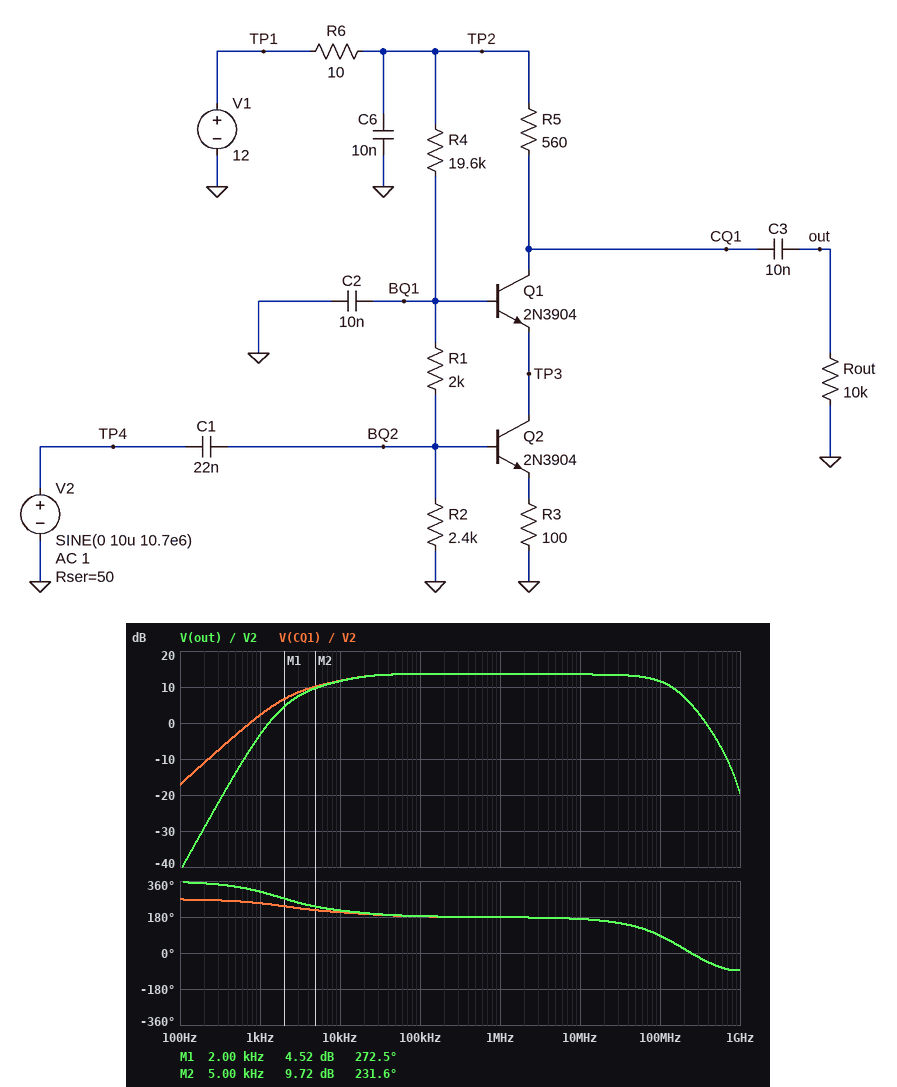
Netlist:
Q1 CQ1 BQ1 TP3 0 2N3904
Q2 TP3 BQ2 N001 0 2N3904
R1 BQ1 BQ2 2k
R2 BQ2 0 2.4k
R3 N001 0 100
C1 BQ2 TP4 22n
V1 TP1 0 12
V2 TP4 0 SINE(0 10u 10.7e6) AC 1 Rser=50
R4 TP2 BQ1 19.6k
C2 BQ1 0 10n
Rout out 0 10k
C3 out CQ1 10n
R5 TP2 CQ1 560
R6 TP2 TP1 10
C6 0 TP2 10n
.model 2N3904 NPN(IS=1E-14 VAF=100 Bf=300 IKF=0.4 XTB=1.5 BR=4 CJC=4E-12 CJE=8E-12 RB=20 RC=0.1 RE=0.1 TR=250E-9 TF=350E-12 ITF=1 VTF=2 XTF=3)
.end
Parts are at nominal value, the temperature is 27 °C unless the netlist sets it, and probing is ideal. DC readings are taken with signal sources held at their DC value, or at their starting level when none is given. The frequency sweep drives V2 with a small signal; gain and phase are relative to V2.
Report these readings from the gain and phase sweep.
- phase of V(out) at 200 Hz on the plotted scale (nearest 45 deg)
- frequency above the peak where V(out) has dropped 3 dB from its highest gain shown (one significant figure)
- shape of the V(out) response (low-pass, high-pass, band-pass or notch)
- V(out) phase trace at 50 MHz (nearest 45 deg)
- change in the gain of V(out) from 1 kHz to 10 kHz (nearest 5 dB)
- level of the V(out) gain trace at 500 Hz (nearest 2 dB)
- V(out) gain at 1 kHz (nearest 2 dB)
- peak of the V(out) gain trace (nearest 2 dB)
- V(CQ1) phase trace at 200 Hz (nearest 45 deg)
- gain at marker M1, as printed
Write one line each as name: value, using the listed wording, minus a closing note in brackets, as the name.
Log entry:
phase of V(out) at 200 Hz on the plotted scale: 360 deg
frequency above the peak where V(out) has dropped 3 dB from its highest gain shown: 100 MHz
shape of the V(out) response: band-pass
V(out) phase trace at 50 MHz: 135 deg
change in the gain of V(out) from 1 kHz to 10 kHz: 15 dB
level of the V(out) gain trace at 500 Hz: -14 dB
V(out) gain at 1 kHz: -4 dB
peak of the V(out) gain trace: 14 dB
V(CQ1) phase trace at 200 Hz: 270 deg
gain at marker M1, as printed: 4.52 dB
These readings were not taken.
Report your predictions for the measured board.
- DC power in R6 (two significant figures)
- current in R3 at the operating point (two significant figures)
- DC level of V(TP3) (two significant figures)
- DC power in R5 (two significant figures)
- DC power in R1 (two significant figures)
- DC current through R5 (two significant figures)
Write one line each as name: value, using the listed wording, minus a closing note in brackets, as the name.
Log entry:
DC power in R6: 240 µW
current in R3 at the operating point: 4.4 mA
DC level of V(TP3): 1.4 V
DC power in R5: 11 mW
DC power in R1: 480 µW
DC current through R5: 4.4 mA
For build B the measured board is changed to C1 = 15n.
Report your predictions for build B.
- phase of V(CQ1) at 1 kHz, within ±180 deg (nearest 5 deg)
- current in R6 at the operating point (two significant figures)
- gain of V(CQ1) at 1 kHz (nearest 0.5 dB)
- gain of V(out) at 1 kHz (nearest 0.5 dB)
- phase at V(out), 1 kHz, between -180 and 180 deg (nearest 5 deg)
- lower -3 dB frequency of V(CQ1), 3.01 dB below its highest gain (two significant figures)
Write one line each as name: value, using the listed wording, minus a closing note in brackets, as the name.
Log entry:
phase of V(CQ1) at 1 kHz, within ±180 deg: -105 deg
current in R6 at the operating point: 4.9 mA
gain of V(CQ1) at 1 kHz: -1.0 dB
gain of V(out) at 1 kHz: -6.5 dB
phase at V(out), 1 kHz, between -180 and 180 deg: -50 deg
lower -3 dB frequency of V(CQ1), 3.01 dB below its highest gain: 10 kHz
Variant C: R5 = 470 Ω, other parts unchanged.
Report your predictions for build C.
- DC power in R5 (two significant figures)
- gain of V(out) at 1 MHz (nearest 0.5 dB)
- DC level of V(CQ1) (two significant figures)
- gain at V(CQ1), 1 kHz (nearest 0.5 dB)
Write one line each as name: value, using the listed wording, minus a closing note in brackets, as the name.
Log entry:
DC power in R5: 9.1 mW
gain of V(out) at 1 MHz: 12.0 dB
DC level of V(CQ1): 9.9 V
gain at V(CQ1), 1 kHz: 0.5 dB
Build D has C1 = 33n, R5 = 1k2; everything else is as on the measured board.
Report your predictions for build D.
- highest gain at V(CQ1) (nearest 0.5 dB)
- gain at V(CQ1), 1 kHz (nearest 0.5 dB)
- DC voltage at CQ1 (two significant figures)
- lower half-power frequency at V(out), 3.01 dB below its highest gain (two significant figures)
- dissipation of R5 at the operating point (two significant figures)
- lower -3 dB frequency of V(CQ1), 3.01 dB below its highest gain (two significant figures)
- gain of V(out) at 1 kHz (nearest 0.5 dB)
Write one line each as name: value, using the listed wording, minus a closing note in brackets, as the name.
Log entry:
highest gain at V(CQ1): 19.5 dB
gain at V(CQ1), 1 kHz: 11.5 dB
DC voltage at CQ1: 6.7 V
lower half-power frequency at V(out), 3.01 dB below its highest gain: 4.2 kHz
dissipation of R5 at the operating point: 23 mW
lower -3 dB frequency of V(CQ1), 3.01 dB below its highest gain: 3.1 kHz
gain of V(out) at 1 kHz: 6.0 dB
